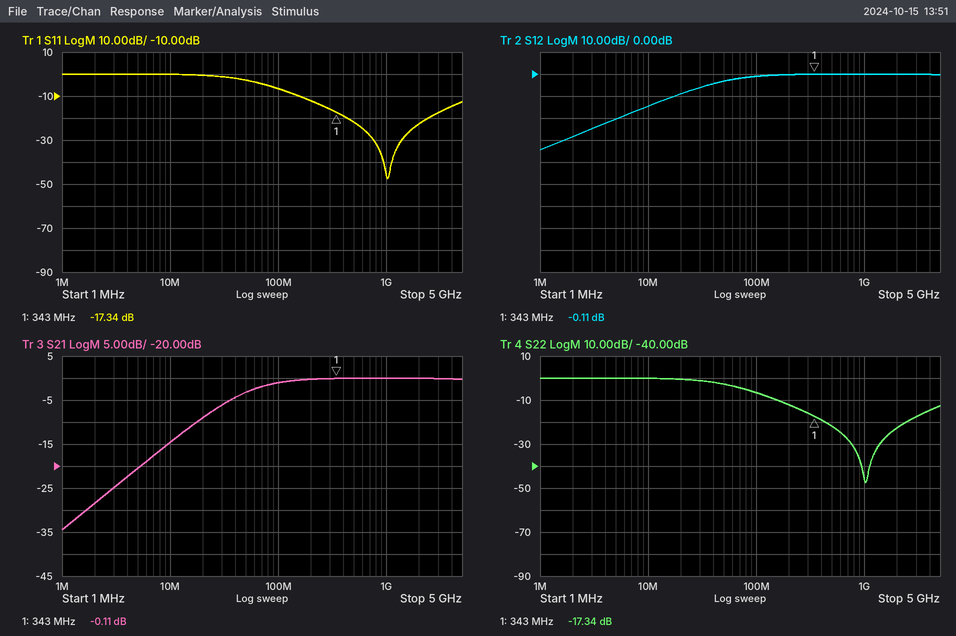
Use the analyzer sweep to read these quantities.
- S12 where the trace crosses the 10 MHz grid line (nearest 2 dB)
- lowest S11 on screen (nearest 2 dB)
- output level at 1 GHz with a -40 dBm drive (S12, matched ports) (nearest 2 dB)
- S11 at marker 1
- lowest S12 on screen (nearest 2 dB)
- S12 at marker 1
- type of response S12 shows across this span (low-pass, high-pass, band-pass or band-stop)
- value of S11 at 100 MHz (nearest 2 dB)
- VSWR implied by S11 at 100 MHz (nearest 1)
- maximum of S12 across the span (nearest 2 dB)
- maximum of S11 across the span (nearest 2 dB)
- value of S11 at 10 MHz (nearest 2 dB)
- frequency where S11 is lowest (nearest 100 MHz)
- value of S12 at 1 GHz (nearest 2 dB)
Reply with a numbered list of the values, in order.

1. -14 dB
2. -48 dB
3. -40 dBm
4. -17.34 dB
5. -34 dB
6. -0.11 dB
7. high-pass
8. -6 dB
9. 3
10. 0 dB
11. 0 dB
12. 0 dB
13. 1.0 GHz
14. 0 dB
